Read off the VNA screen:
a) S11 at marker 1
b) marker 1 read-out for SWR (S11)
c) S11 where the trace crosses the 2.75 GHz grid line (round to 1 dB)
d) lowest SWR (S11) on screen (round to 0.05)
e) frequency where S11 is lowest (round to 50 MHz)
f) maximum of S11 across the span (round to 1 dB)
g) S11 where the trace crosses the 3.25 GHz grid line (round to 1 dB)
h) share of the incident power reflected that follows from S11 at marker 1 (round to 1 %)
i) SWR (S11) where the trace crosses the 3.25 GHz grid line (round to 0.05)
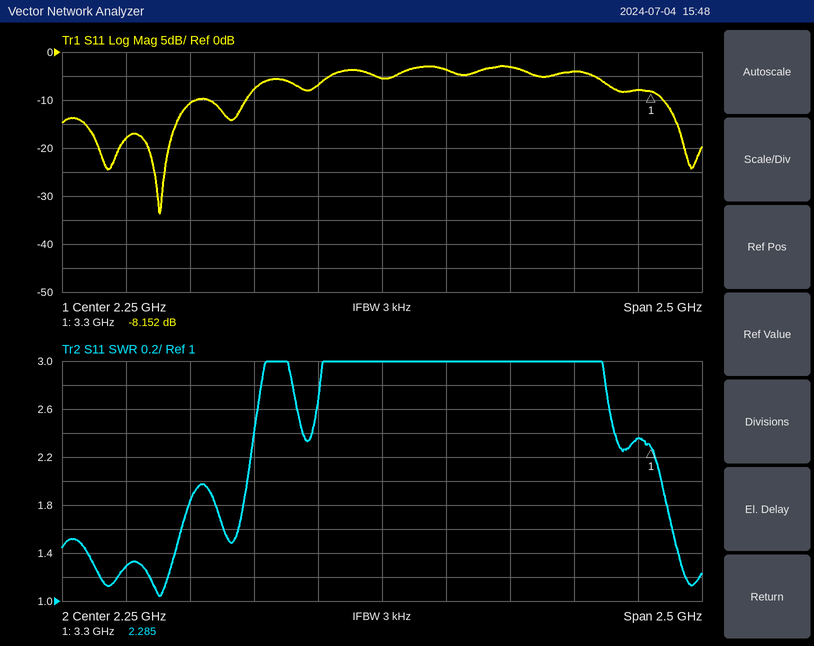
-8.152 dB
2.285
-3 dB
1.05
1.40 GHz
-3 dB
-8 dB
15 %
2.35
